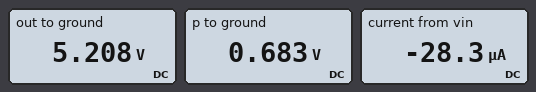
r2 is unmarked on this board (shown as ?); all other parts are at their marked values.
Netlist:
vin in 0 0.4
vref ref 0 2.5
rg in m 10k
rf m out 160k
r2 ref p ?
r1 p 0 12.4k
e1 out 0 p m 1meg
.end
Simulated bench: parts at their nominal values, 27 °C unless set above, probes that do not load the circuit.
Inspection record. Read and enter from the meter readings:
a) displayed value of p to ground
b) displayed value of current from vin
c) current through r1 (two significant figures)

0.683 V
-28.3 µA
55 µA
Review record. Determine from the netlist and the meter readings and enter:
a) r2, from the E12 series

33 kΩ
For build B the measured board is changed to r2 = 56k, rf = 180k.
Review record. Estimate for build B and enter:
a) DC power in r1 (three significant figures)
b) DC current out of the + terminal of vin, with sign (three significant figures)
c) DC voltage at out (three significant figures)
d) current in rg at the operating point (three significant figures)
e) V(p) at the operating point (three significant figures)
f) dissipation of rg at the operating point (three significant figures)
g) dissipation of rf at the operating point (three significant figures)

16.6 µW
-5.32 µA
1.41 V
5.32 µA
453 mV
283 nW
5.10 µW
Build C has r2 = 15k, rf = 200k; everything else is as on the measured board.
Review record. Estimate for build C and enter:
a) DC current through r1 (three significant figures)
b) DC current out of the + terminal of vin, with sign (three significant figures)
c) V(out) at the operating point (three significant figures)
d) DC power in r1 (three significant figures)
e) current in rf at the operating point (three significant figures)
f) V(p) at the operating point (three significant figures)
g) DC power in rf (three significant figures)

91.2 µA
-73.1 µA
15.8 V
103 µW
73.1 µA
1.13 V
1.07 mW
